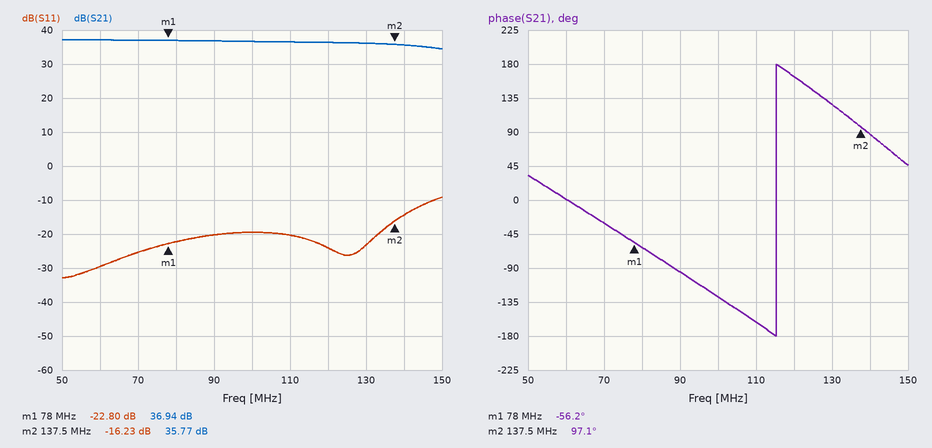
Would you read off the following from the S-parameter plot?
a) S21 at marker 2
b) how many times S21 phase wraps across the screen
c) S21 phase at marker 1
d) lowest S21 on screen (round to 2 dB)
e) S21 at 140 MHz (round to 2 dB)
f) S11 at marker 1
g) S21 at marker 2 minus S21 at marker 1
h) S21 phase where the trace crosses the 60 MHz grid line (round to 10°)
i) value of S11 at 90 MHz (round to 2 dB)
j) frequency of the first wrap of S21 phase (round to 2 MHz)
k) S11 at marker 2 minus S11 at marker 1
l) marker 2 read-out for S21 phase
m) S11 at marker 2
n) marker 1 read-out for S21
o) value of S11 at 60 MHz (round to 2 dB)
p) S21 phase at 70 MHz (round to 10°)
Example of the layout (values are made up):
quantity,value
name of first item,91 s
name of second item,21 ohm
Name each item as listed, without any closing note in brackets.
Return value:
quantity,value
S21 at marker 2,35.77 dB
how many times S21 phase wraps across the screen,1
S21 phase at marker 1,-56.2°
lowest S21 on screen,34 dB
S21 at 140 MHz,36 dB
S11 at marker 1,-22.80 dB
S21 at marker 2 minus S21 at marker 1,-1.17 dB
S21 phase where the trace crosses the 60 MHz grid line,0°
value of S11 at 90 MHz,-20 dB
frequency of the first wrap of S21 phase,116 MHz
S11 at marker 2 minus S11 at marker 1,6.57 dB
marker 2 read-out for S21 phase,97.1°
S11 at marker 2,-16.23 dB
marker 1 read-out for S21,36.94 dB
value of S11 at 60 MHz,-30 dB
S21 phase at 70 MHz,-30°
